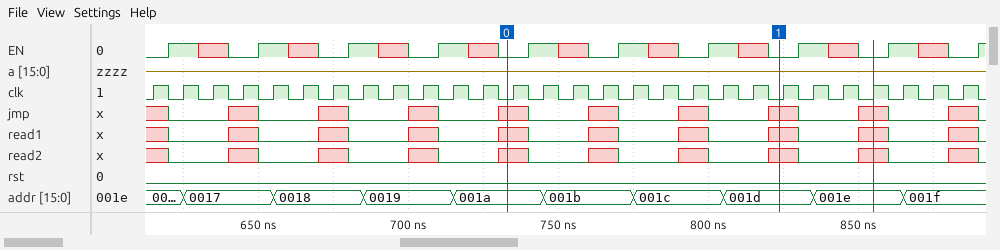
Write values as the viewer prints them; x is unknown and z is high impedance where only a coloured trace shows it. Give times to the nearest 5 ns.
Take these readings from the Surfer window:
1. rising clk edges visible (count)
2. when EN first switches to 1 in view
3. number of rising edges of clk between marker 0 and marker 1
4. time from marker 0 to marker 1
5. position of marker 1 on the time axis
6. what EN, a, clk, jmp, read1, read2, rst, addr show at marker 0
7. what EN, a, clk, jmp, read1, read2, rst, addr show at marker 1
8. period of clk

28
620 ns
9
90 ns
825 ns
EN=0, a=z, clk=0, jmp=x, read1=x, read2=x, rst=0, addr=001a
EN=0, a=z, clk=0, jmp=x, read1=x, read2=x, rst=0, addr=001d
10 ns
